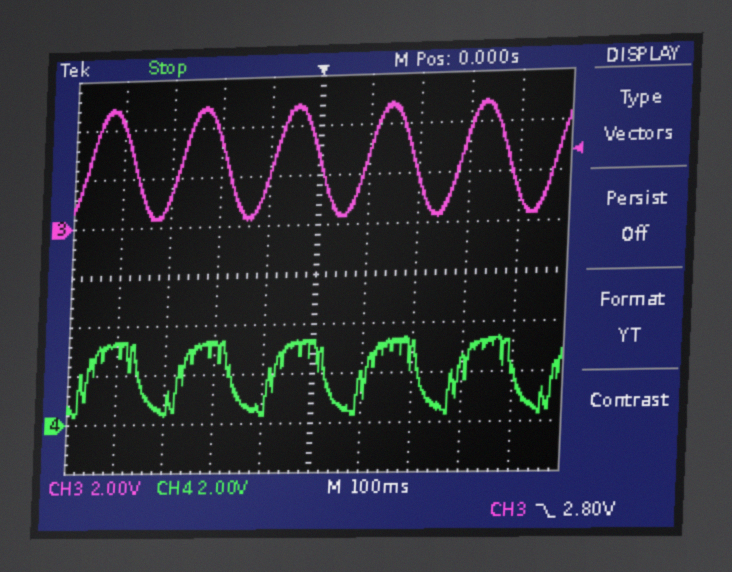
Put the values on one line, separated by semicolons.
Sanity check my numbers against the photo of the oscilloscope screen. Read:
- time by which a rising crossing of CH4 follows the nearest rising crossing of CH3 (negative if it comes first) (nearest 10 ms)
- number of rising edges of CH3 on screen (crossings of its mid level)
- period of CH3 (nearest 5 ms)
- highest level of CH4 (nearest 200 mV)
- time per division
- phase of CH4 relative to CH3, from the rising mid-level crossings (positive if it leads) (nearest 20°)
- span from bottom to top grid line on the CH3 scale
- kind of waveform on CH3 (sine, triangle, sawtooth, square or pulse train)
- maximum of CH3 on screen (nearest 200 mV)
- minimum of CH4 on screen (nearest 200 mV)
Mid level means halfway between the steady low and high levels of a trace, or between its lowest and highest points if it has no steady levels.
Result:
+10 ms; 6; 190 ms; 3.4 V; 100 ms; -20°; 16 V; sine; 4.8 V; 400 mV
